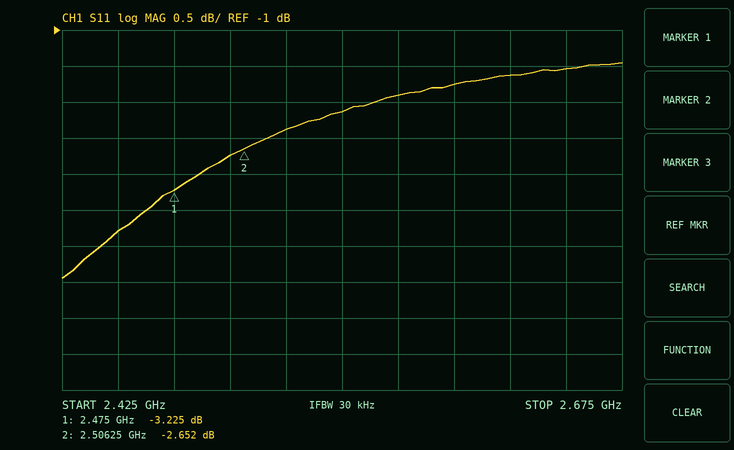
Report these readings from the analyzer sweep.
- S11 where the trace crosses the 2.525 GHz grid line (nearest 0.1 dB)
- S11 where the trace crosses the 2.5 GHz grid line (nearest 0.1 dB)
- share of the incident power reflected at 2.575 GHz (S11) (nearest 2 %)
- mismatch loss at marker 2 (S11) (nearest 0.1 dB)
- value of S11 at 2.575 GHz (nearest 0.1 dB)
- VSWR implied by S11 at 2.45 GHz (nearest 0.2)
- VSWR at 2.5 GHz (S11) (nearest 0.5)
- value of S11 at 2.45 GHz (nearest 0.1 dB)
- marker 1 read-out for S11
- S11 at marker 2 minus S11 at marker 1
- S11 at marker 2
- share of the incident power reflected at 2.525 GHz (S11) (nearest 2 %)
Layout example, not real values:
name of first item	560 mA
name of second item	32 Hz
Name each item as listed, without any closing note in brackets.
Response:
S11 where the trace crosses the 2.525 GHz grid line	-2.4 dB
S11 where the trace crosses the 2.5 GHz grid line	-2.7 dB
share of the incident power reflected at 2.575 GHz (S11)	64 %
mismatch loss at marker 2 (S11)	3.4 dB
value of S11 at 2.575 GHz	-1.9 dB
VSWR implied by S11 at 2.45 GHz	4.6
VSWR at 2.5 GHz (S11)	6.5
value of S11 at 2.45 GHz	-3.8 dB
marker 1 read-out for S11	-3.225 dB
S11 at marker 2 minus S11 at marker 1	0.573 dB
S11 at marker 2	-2.652 dB
share of the incident power reflected at 2.525 GHz (S11)	58 %
